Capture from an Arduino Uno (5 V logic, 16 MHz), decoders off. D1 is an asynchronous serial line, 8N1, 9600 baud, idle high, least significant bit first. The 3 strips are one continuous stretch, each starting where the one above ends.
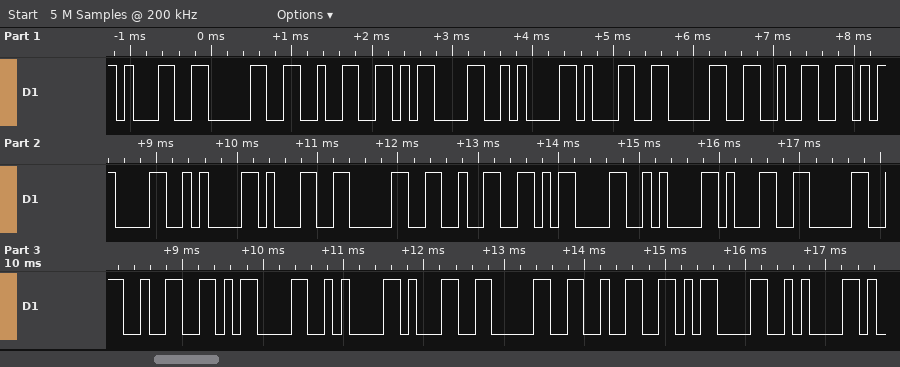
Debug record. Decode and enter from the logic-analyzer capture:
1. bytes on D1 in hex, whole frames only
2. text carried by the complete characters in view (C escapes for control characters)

31 30 32 0D 0A 31 30 32 0D 0A 31 30 32 0D 0A 31 30 32 0D 0A 31 30 32 0D 0A
"102\r\n102\r\n102\r\n102\r\n102\r\n"
